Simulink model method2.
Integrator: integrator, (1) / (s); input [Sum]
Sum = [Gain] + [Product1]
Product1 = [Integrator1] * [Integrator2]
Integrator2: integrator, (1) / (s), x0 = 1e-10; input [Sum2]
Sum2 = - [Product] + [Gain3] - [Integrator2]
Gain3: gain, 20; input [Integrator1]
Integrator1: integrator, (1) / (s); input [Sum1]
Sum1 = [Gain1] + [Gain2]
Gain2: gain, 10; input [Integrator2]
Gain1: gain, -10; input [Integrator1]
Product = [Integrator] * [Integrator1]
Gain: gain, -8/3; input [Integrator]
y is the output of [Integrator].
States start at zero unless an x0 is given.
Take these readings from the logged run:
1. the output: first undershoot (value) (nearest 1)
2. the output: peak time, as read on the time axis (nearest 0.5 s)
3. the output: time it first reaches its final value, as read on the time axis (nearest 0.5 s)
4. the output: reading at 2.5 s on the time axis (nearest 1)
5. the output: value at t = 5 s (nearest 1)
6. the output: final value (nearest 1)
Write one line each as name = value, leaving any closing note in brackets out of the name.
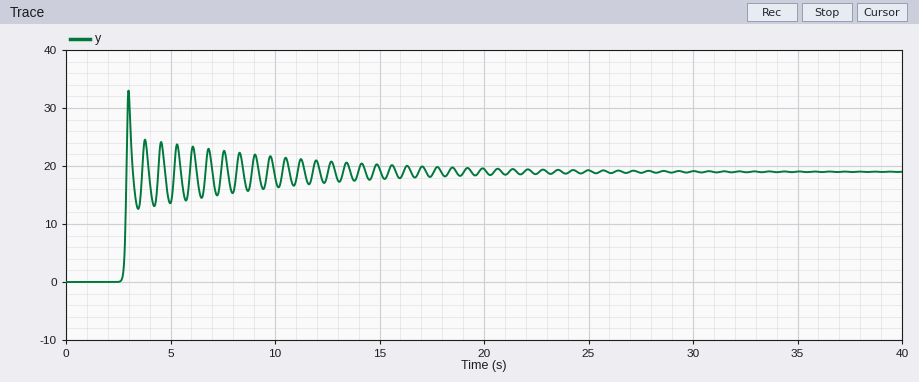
the output: first undershoot (value) = 13
the output: peak time, as read on the time axis = 3.0 s
the output: time it first reaches its final value, as read on the time axis = 3.0 s
the output: reading at 2.5 s on the time axis = 0
the output: value at t = 5 s = 14
the output: final value = 19
